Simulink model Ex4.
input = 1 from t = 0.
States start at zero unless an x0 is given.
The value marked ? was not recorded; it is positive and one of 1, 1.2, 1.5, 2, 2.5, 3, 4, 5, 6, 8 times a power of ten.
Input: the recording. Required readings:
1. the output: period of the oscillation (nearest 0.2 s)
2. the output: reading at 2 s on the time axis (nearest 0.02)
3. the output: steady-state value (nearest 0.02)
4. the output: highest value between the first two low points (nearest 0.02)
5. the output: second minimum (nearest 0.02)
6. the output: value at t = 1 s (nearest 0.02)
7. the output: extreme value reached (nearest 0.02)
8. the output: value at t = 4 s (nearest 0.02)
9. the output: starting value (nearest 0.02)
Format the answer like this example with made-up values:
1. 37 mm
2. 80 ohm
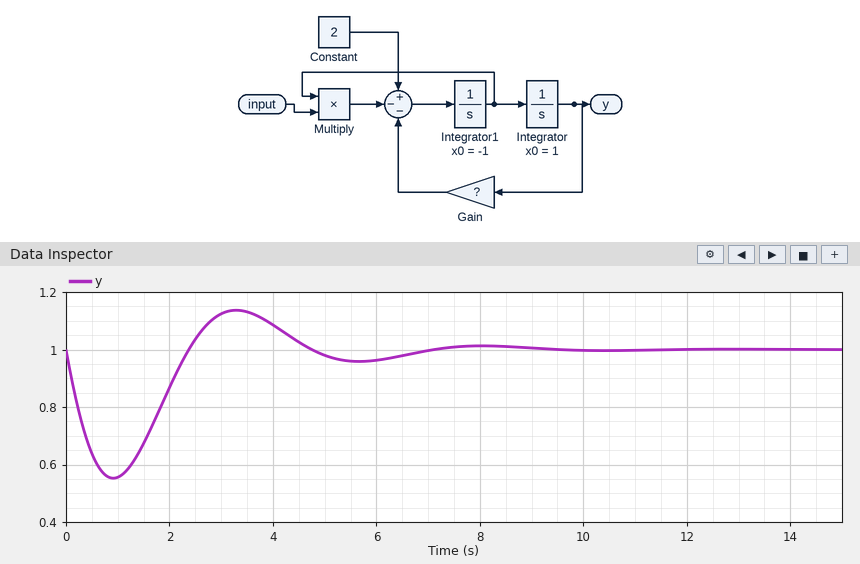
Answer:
1. 4.8 s
2. 0.86
3. 1.00
4. 1.14
5. 0.96
6. 0.56
7. 0.56
8. 1.08
9. 1.00
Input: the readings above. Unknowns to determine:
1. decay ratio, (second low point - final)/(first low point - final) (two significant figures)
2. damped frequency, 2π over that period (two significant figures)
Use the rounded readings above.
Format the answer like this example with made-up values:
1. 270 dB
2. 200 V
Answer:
1. 0.091
2. 1.3 rad/s
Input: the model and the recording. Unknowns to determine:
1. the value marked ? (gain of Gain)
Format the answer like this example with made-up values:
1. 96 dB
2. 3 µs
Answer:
1. 2
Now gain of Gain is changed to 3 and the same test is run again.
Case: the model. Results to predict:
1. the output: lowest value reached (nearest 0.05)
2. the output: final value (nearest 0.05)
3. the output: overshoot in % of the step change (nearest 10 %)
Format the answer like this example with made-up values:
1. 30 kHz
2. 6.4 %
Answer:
1. 0.35
2. 0.65
3. 100 %
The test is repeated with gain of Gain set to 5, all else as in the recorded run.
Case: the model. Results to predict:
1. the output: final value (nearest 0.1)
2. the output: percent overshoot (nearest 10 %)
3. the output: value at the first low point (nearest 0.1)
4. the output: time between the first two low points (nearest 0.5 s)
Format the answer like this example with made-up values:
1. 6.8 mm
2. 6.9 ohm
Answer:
1. 0.4
2. 60 %
3. 0.0
4. 3.0 s
